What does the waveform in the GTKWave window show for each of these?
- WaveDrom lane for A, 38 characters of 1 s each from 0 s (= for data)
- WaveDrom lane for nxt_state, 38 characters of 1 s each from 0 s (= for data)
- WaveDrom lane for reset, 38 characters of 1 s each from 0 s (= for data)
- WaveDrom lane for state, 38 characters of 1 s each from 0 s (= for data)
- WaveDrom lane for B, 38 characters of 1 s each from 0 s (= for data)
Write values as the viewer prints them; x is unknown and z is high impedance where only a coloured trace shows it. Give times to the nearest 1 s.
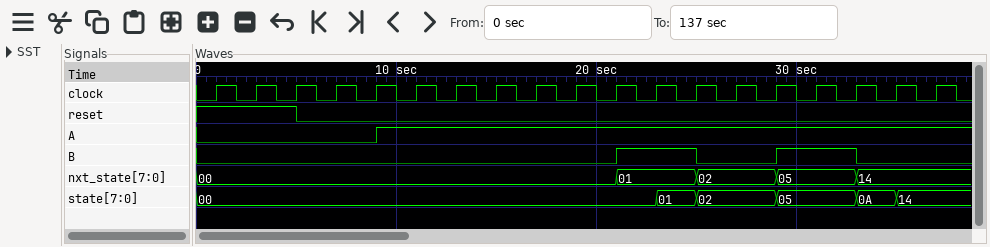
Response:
{name: 'A', wave: '0........1............................'}
{name: 'nxt_state', wave: '=....................=...=...=...=....', data: '00 01 02 05 14'}
{name: 'reset', wave: '1....0................................'}
{name: 'state', wave: '=......................=.=...=...=.=..', data: '00 01 02 05 0A 14'}
{name: 'B', wave: '0....................1...0...1...0....'}
